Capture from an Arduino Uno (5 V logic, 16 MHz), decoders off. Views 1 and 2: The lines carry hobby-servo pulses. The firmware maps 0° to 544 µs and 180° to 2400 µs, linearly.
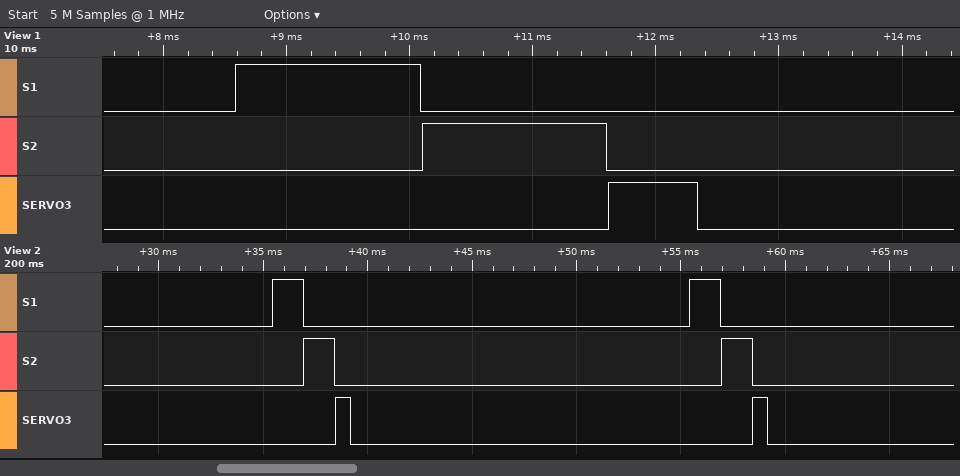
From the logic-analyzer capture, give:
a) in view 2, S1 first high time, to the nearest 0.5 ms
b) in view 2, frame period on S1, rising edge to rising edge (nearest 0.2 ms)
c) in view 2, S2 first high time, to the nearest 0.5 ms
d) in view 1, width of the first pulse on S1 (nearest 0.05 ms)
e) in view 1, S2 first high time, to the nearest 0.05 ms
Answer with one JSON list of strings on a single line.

["1.5 ms", "20.0 ms", "1.5 ms", "1.50 ms", "1.50 ms"]
